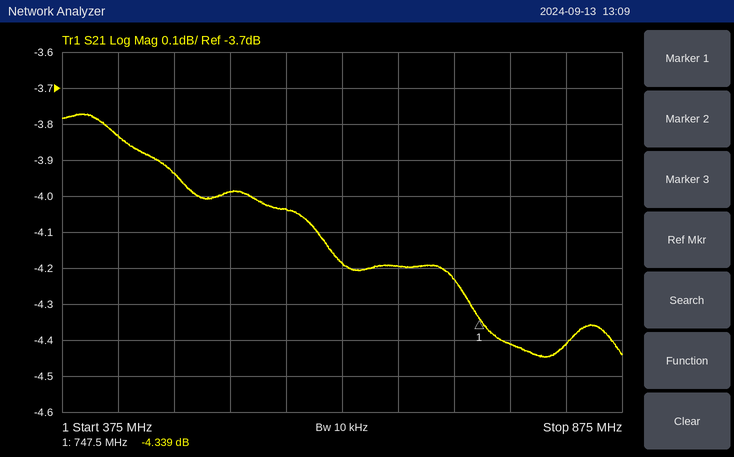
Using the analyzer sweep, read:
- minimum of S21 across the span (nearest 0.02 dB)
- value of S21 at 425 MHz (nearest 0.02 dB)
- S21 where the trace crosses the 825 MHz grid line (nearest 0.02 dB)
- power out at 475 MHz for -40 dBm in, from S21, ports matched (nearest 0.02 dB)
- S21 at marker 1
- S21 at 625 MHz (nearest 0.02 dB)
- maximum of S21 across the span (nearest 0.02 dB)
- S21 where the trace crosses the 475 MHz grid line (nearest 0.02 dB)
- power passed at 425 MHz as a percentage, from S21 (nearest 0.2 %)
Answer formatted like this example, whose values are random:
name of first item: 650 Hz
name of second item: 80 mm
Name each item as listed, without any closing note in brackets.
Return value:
minimum of S21 across the span: -4.44 dB
value of S21 at 425 MHz: -3.84 dB
S21 where the trace crosses the 825 MHz grid line: -4.42 dB
power out at 475 MHz for -40 dBm in, from S21, ports matched: -43.94 dBm
S21 at marker 1: -4.339 dB
S21 at 625 MHz: -4.18 dB
maximum of S21 across the span: -3.78 dB
S21 where the trace crosses the 475 MHz grid line: -3.94 dB
power passed at 425 MHz as a percentage, from S21: 41.4 %
